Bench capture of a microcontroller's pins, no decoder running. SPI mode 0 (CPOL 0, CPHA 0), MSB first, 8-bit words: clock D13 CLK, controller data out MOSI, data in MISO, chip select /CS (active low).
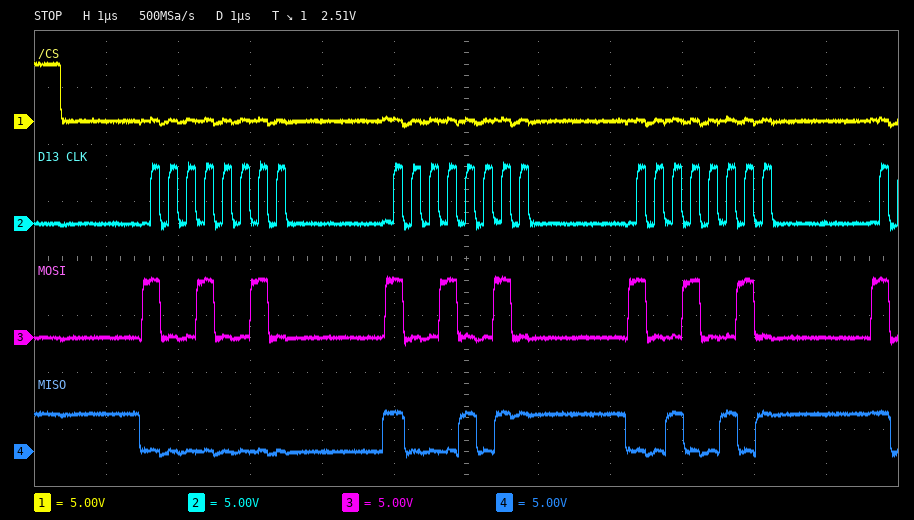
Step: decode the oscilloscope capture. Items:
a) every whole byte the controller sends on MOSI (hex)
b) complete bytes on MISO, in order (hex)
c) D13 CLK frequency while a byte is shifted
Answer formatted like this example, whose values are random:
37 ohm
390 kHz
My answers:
92 92 92
00 8B 25
4 MHz
